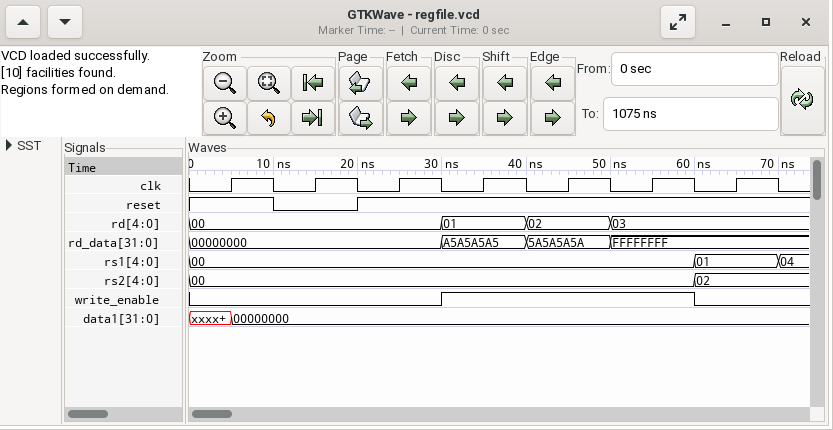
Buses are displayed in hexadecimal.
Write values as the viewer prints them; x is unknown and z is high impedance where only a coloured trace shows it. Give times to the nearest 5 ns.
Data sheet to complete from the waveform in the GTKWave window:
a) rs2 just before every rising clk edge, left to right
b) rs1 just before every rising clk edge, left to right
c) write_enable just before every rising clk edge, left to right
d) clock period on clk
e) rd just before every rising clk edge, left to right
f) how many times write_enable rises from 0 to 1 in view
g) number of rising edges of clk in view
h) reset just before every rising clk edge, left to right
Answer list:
00, 00, 00, 00, 00, 00, 02
00, 00, 00, 00, 00, 00, 01
0 0 0 1 1 1 0
10 ns
00, 00, 00, 01, 02, 03, 03
1
7
1 0 1 1 1 1 1
